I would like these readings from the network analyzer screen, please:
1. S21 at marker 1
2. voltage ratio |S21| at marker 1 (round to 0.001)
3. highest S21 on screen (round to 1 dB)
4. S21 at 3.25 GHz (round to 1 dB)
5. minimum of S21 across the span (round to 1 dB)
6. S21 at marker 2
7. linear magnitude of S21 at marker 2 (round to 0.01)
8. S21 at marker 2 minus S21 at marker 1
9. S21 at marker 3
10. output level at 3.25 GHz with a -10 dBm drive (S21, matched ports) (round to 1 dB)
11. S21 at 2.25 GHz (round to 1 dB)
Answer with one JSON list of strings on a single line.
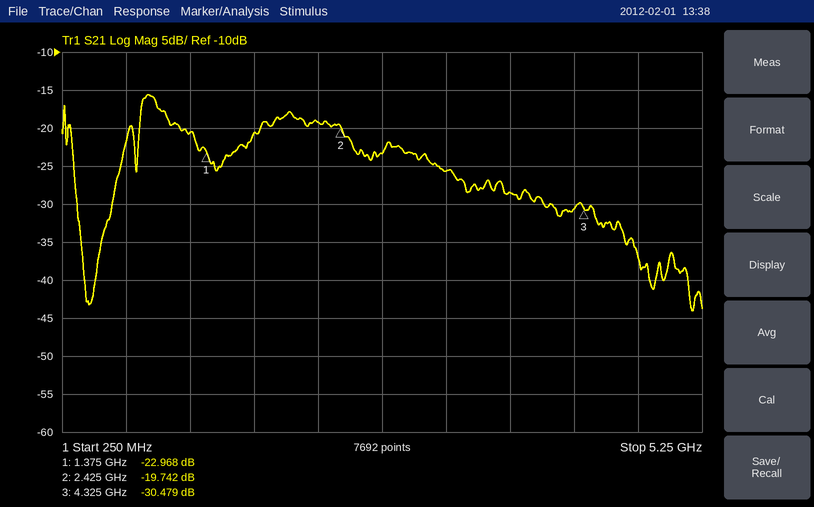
["-22.968 dB", "0.071", "-16 dB", "-26 dB", "-44 dB", "-19.742 dB", "0.10", "3.226 dB", "-30.479 dB", "-36 dBm", "-19 dB"]
